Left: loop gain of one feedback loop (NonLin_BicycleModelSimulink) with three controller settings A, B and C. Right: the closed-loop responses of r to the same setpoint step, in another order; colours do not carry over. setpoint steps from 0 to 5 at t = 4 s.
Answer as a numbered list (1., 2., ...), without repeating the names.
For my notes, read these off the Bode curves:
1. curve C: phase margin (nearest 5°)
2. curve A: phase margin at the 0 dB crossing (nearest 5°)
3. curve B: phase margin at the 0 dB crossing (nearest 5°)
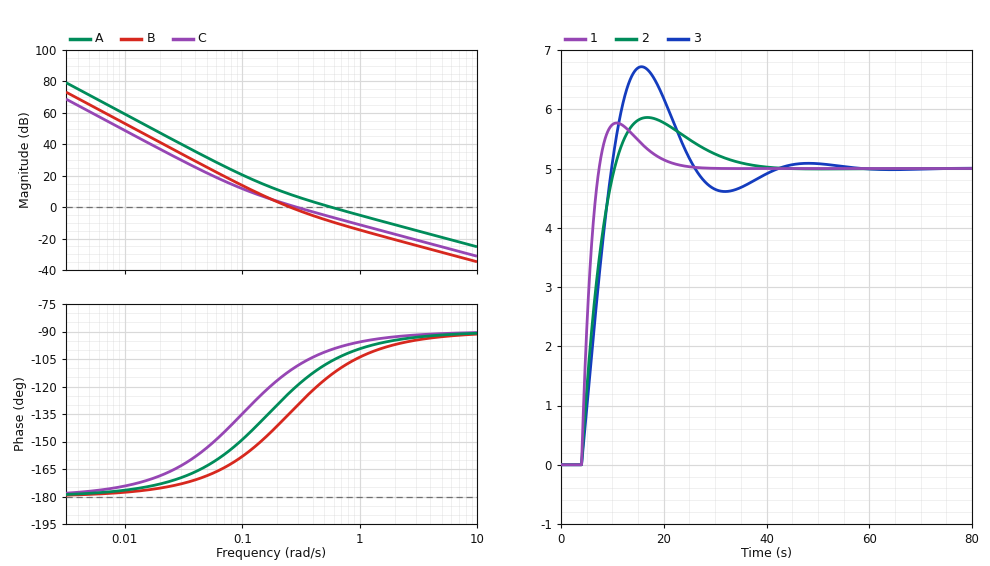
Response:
1. 70°
2. 75°
3. 45°
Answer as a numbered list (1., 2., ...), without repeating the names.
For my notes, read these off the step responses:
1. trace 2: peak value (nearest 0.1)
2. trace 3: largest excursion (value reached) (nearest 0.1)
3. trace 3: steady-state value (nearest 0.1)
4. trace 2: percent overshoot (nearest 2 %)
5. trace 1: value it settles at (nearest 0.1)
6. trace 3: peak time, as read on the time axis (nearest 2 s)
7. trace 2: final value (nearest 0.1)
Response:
1. 5.9
2. 6.7
3. 5.0
4. 18 %
5. 5.0
6. 16 s
7. 5.0
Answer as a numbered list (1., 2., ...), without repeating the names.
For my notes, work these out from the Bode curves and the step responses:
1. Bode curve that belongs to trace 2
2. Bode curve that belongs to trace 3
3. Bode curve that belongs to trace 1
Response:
1. C
2. B
3. A
